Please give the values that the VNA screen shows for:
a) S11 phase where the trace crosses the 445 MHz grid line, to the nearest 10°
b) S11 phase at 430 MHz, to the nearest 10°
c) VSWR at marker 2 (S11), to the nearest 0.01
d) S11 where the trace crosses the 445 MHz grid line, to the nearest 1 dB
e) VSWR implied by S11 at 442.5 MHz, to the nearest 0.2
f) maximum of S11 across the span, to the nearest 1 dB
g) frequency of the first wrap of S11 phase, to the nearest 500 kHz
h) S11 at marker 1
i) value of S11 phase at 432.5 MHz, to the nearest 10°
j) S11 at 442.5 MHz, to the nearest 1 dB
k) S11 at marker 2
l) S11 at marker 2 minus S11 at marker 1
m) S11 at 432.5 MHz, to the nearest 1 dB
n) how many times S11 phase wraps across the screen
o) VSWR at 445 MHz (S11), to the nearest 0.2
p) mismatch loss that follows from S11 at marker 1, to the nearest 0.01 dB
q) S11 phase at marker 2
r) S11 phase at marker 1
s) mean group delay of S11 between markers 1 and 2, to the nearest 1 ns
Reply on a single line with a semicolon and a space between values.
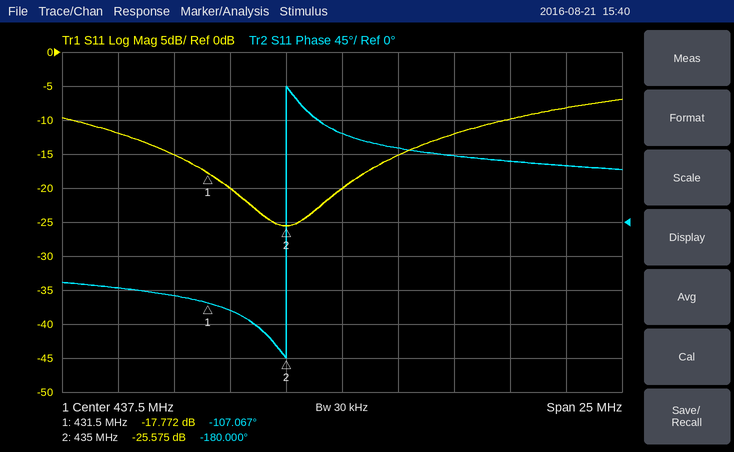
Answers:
80°; -100°; 1.11; -10 dB; 1.6; -7 dB; 435.0 MHz; -17.772 dB; -120°; -12 dB; -25.575 dB; -7.803 dB; -20 dB; 1; 2.0; 0.07 dB; -180.000°; -107.067°; 58 ns
